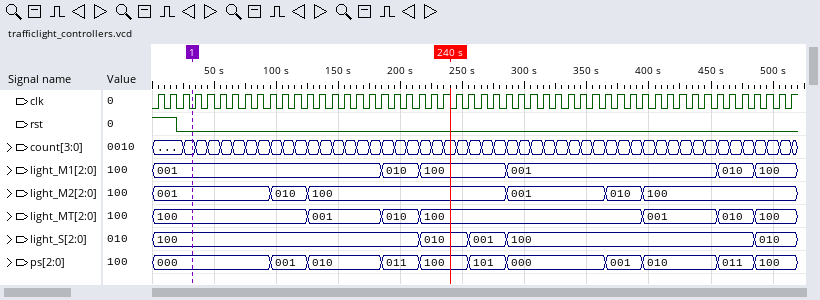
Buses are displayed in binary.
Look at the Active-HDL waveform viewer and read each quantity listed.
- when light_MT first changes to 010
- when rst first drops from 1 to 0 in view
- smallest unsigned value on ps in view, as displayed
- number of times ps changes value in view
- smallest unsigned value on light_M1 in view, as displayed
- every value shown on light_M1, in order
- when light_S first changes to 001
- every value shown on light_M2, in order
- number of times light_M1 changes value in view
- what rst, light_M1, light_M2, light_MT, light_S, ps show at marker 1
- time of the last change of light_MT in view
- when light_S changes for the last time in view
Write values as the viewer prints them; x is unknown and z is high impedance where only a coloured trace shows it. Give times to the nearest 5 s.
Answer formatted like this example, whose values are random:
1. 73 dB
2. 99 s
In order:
1. 185 s
2. 20 s
3. 000
4. 10
5. 001
6. 001, 010, 100, 001, 010, 100
7. 255 s
8. 001, 010, 100, 001, 010, 100
9. 5
10. rst=0, light_M1=001, light_M2=001, light_MT=100, light_S=100, ps=000
11. 485 s
12. 485 s
